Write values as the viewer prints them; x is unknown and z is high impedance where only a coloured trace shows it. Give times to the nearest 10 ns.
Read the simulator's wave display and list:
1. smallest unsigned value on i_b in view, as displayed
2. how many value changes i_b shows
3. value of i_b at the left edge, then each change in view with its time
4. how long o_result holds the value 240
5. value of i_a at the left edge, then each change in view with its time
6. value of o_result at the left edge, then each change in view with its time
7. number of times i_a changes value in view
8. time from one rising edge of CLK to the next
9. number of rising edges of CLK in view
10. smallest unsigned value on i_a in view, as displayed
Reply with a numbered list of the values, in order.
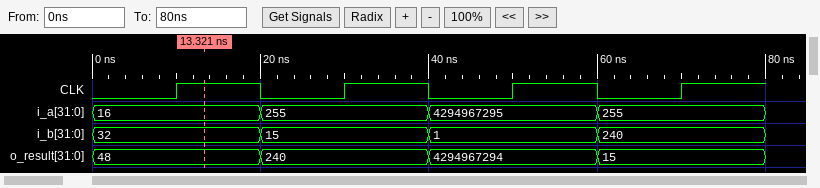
1. 1
2. 3
3. 32, 15 at 20 ns, 1 at 40 ns, 240 at 60 ns
4. 20 ns
5. 16, 255 at 20 ns, 4294967295 at 40 ns, 255 at 60 ns
6. 48, 240 at 20 ns, 4294967294 at 40 ns, 15 at 60 ns
7. 3
8. 20 ns
9. 4
10. 16
